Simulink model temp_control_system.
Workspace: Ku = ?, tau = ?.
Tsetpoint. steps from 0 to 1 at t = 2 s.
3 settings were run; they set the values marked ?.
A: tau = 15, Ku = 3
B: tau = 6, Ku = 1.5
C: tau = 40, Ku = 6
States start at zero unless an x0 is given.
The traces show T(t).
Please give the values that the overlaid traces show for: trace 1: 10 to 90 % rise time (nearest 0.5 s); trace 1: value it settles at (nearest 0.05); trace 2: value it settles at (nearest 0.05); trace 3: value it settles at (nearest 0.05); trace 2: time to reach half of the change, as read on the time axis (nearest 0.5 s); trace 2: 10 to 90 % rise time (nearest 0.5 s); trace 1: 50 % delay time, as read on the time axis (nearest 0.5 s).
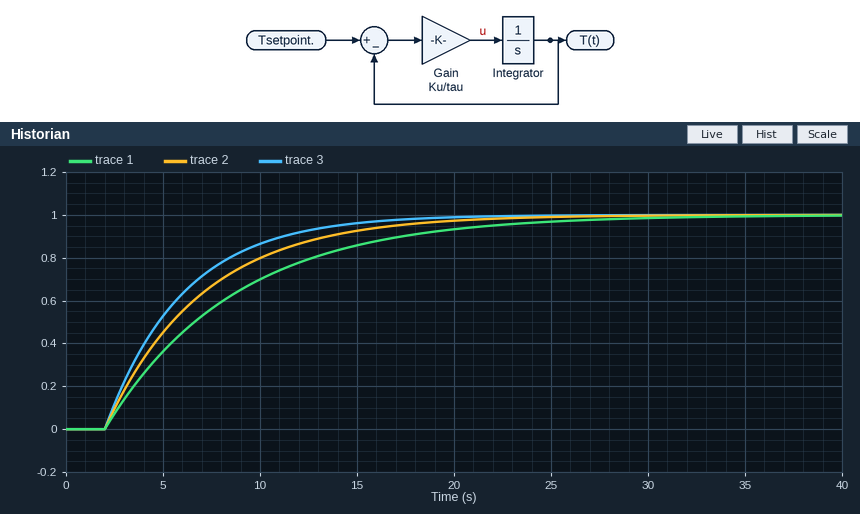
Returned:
14.5 s
1.00
1.00
1.00
5.5 s
11.0 s
6.5 s
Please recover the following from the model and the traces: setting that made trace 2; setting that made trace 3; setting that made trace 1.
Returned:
A
B
C
